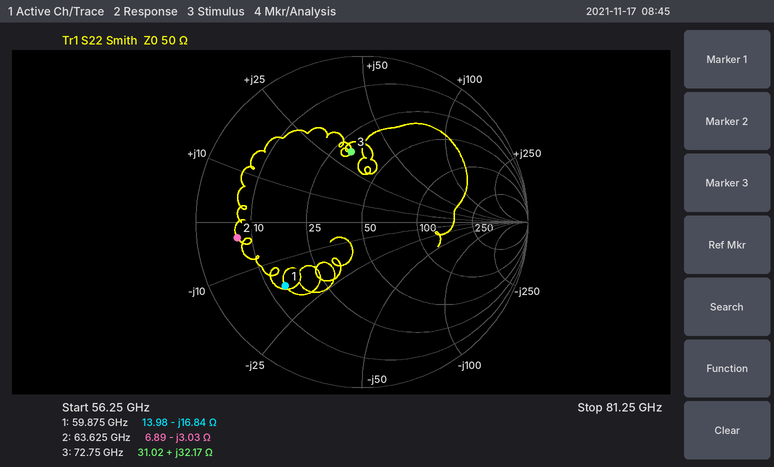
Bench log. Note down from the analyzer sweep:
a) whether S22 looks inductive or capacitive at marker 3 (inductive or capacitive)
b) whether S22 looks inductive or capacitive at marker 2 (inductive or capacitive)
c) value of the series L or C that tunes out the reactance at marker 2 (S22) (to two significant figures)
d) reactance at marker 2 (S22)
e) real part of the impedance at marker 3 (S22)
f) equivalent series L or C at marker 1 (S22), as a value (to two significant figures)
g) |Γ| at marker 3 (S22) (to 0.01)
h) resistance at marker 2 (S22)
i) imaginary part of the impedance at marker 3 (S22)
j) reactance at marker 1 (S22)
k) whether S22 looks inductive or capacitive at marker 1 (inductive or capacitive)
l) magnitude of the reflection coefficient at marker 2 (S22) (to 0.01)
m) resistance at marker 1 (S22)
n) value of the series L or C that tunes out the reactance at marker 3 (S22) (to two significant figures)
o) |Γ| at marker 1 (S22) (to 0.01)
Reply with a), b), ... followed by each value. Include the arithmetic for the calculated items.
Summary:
a) inductive
b) capacitive
c) L = 3.03 Ω/(2π × 63.625 GHz) ≈ 7.6 pH
d) -3.03 Ω
e) 31.02 Ω
f) C = 1/(2π × 59.875 GHz × 16.84 Ω) ≈ 158 fF, so 160 fF to two significant figures
g) 0.43
h) 6.89 Ω
i) +32.17 Ω
j) -16.84 Ω
k) capacitive
l) 0.76
m) 13.98 Ω
n) C = 1/(2π × 72.75 GHz × 32.17 Ω) ≈ 68 fF
o) 0.60
